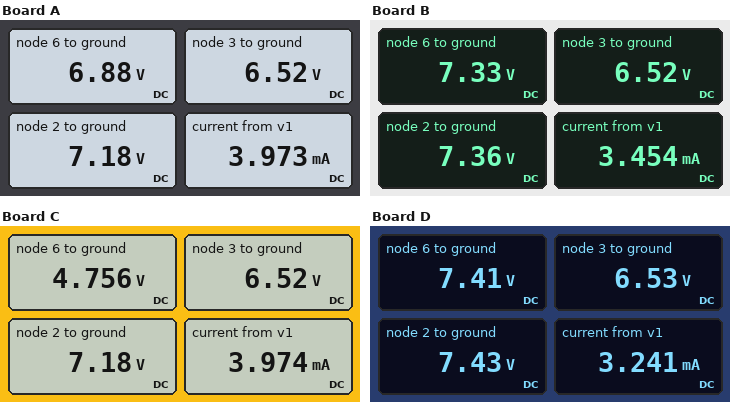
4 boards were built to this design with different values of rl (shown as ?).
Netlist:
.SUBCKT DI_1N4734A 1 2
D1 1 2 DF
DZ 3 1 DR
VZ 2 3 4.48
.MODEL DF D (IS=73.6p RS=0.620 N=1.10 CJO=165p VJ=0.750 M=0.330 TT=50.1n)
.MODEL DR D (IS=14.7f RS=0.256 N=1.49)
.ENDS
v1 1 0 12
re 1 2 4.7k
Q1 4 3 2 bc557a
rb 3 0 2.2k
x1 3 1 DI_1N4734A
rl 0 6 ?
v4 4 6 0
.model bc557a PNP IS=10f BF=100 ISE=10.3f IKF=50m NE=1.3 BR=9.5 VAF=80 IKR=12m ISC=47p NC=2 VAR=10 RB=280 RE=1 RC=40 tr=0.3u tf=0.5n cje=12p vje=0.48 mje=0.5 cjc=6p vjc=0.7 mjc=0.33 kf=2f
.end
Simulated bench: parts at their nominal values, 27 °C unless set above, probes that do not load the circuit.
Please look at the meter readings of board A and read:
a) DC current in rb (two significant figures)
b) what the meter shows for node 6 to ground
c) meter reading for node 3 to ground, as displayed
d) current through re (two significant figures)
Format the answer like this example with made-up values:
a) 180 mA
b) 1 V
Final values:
a) 3.0 mA
b) 6.88 V
c) 6.52 V
d) 1.0 mA
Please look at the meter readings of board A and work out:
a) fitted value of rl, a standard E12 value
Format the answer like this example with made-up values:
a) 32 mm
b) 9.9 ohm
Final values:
a) 6.8 kΩ
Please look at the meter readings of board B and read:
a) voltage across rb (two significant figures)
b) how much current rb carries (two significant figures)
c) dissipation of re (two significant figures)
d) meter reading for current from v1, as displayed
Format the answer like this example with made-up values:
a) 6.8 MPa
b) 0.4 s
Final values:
a) 6.5 V
b) 3.0 mA
c) 4.6 mW
d) 3.454 mA
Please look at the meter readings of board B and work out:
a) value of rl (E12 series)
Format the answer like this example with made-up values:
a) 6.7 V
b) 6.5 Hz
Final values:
a) 15 kΩ
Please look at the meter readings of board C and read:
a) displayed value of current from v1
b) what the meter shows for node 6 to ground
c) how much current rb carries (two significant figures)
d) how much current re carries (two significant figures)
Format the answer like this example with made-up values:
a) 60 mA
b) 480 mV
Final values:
a) 3.974 mA
b) 4.756 V
c) 3.0 mA
d) 1.0 mA
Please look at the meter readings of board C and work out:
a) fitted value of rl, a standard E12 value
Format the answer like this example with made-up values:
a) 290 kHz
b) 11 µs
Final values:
a) 4.7 kΩ
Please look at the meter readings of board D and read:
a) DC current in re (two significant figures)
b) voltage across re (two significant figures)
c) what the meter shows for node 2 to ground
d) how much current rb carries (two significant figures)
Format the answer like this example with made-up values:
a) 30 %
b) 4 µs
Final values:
a) 970 µA
b) 4.6 V
c) 7.43 V
d) 3.0 mA
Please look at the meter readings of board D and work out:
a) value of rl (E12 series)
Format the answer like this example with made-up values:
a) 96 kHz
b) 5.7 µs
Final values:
a) 27 kΩ
